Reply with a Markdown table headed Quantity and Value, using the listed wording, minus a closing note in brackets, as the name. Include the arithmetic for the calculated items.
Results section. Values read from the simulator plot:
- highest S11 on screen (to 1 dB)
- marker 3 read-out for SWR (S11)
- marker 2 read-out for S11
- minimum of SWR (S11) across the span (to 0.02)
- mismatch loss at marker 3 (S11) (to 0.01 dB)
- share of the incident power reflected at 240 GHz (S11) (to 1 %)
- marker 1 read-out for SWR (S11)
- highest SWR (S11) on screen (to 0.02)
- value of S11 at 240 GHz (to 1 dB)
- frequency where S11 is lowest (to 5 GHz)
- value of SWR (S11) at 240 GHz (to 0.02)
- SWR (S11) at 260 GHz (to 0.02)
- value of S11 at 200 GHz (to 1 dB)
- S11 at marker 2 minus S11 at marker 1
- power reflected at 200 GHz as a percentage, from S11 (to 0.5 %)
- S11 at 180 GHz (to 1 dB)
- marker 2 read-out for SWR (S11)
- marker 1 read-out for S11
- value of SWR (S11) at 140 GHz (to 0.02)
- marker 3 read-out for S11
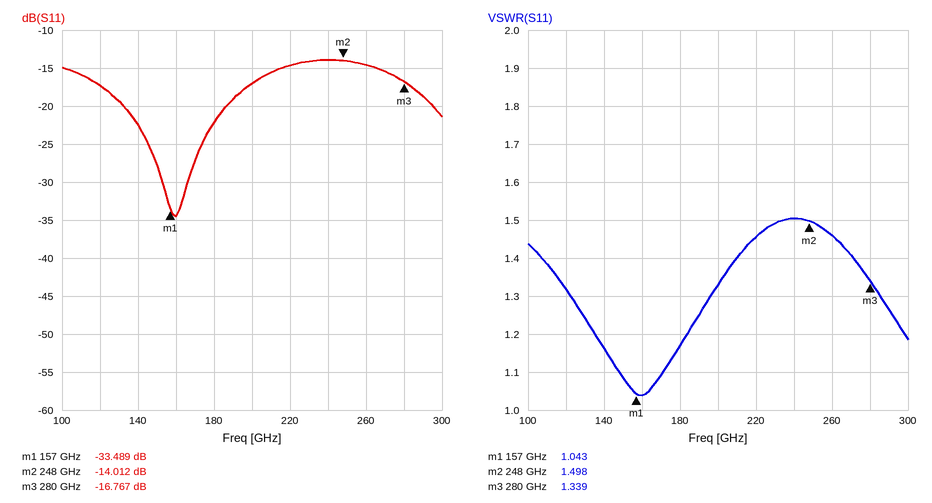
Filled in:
| Quantity | Value |
|---|---|
| highest S11 on screen | -14 dB |
| marker 3 read-out for SWR | 1.339 |
| marker 2 read-out for S11 | -14.012 dB |
| minimum of SWR (S11) across the span | 1.04 |
| mismatch loss at marker 3 (S11) | −10 log10(1 − 10^(-16.767/10)) ≈ 0.09 dB |
| share of the incident power reflected at 240 GHz (S11) | 10^(-14/10) ≈ 4 % |
| marker 1 read-out for SWR | 1.043 |
| highest SWR (S11) on screen | 1.50 |
| value of S11 at 240 GHz | -14 dB |
| frequency where S11 is lowest | 160 GHz |
| value of SWR (S11) at 240 GHz | 1.50 |
| SWR (S11) at 260 GHz | 1.46 |
| value of S11 at 200 GHz | -17 dB |
| S11 at marker 2 minus S11 at marker 1 | -14.012 − (-33.489) = 19.477 dB |
| power reflected at 200 GHz as a percentage, from S11 | 10^(-17/10) ≈ 2.0 % |
| S11 at 180 GHz | -22 dB |
| marker 2 read-out for SWR | 1.498 |
| marker 1 read-out for S11 | -33.489 dB |
| value of SWR (S11) at 140 GHz | 1.16 |
| marker 3 read-out for S11 | -16.767 dB |
